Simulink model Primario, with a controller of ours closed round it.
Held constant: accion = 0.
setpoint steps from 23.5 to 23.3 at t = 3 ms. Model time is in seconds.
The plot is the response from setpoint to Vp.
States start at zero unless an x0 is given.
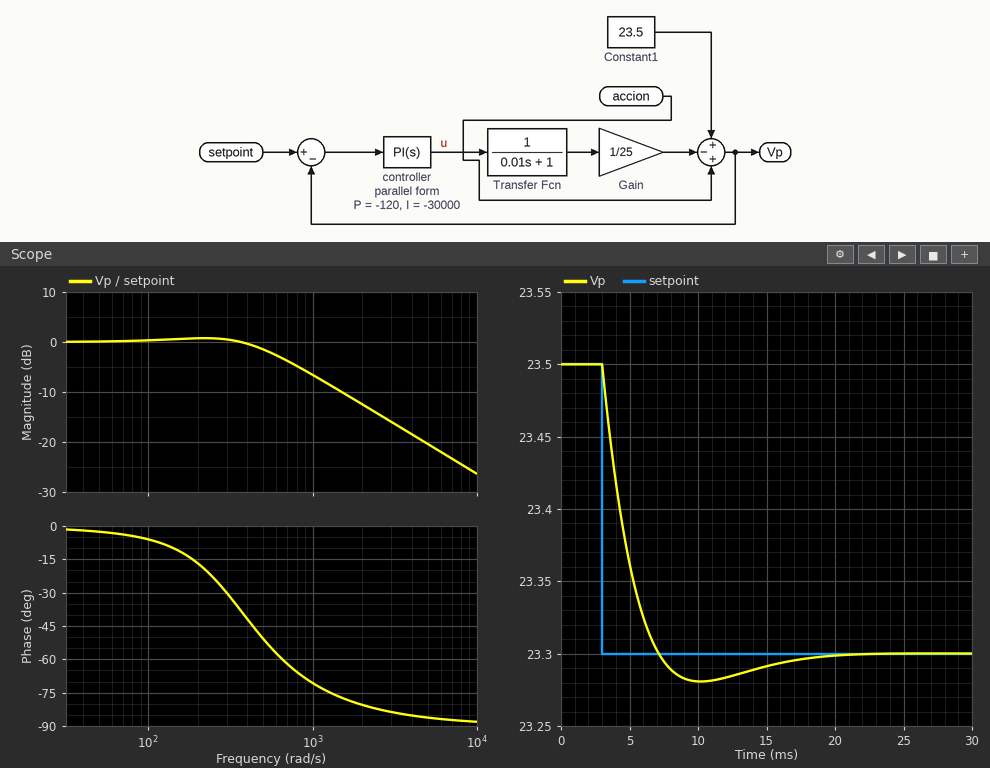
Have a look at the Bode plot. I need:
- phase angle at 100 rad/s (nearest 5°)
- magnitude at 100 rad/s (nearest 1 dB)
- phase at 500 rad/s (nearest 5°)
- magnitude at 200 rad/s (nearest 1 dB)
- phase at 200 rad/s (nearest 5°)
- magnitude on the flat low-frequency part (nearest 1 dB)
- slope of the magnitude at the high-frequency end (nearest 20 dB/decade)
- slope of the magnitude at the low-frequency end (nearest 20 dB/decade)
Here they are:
-5°
0 dB
-50°
1 dB
-15°
0 dB
-20 dB/decade
0 dB/decade
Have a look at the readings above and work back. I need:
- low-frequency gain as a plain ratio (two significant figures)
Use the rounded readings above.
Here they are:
1.0
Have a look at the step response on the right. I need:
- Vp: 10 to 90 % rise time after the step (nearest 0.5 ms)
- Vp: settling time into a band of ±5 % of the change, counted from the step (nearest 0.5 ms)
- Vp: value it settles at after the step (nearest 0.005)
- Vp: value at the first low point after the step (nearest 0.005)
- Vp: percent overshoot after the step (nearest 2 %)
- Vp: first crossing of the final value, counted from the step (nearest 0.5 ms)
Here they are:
3.0 ms
11.5 ms
23.300
23.280
10 %
4.0 ms
